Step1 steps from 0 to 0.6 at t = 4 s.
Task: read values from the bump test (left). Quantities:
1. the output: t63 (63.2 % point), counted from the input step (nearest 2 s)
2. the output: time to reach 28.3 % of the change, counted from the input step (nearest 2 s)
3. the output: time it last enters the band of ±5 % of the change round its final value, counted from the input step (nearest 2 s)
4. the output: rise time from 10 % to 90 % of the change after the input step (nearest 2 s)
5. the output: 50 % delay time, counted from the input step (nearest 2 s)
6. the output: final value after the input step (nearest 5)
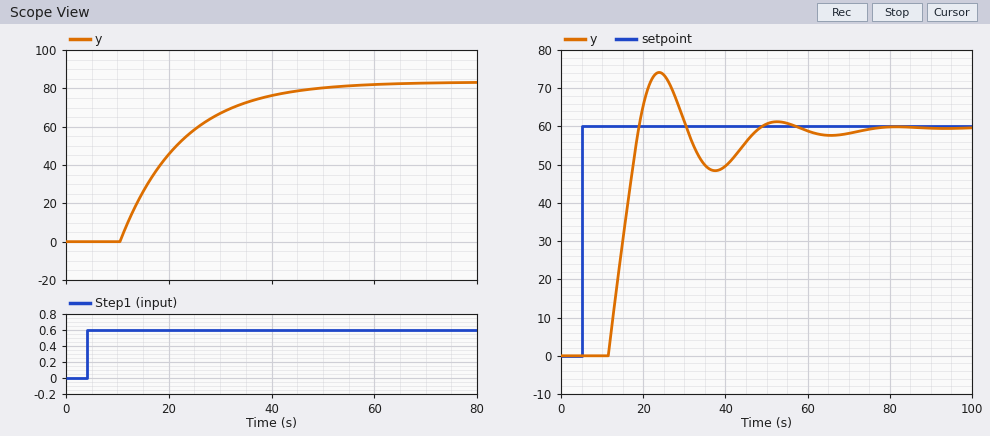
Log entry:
18 s
10 s
42 s
26 s
14 s
85
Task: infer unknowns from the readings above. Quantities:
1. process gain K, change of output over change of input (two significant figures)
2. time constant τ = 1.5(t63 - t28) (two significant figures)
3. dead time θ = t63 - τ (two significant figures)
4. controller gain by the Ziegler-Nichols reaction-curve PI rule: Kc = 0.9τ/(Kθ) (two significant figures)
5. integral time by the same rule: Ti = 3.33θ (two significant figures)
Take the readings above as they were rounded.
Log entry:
140
12 s
6.0 s
0.013
20 s
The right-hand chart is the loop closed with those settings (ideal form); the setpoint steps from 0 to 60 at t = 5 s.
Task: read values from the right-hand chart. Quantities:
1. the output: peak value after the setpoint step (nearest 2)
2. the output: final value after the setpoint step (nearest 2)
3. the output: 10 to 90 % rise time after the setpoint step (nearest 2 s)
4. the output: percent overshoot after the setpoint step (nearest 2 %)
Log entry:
74
60
6 s
24 %
